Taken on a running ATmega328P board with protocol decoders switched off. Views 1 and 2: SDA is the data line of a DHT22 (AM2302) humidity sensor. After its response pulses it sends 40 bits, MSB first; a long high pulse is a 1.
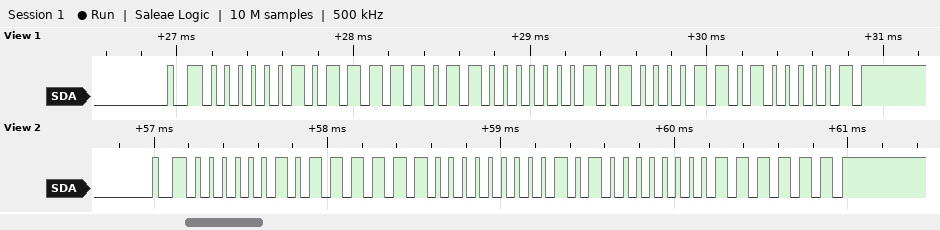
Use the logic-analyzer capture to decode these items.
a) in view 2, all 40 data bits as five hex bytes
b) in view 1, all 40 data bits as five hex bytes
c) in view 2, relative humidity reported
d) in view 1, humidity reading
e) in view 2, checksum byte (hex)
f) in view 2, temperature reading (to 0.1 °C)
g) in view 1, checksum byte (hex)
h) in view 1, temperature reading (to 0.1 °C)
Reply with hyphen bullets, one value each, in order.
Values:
- 02 FC 01 40 3F
- 02 FB 01 43 41
- 76.4 %
- 76.3 %
- 0x3F
- 32.0 °C
- 0x41
- 32.3 °C
